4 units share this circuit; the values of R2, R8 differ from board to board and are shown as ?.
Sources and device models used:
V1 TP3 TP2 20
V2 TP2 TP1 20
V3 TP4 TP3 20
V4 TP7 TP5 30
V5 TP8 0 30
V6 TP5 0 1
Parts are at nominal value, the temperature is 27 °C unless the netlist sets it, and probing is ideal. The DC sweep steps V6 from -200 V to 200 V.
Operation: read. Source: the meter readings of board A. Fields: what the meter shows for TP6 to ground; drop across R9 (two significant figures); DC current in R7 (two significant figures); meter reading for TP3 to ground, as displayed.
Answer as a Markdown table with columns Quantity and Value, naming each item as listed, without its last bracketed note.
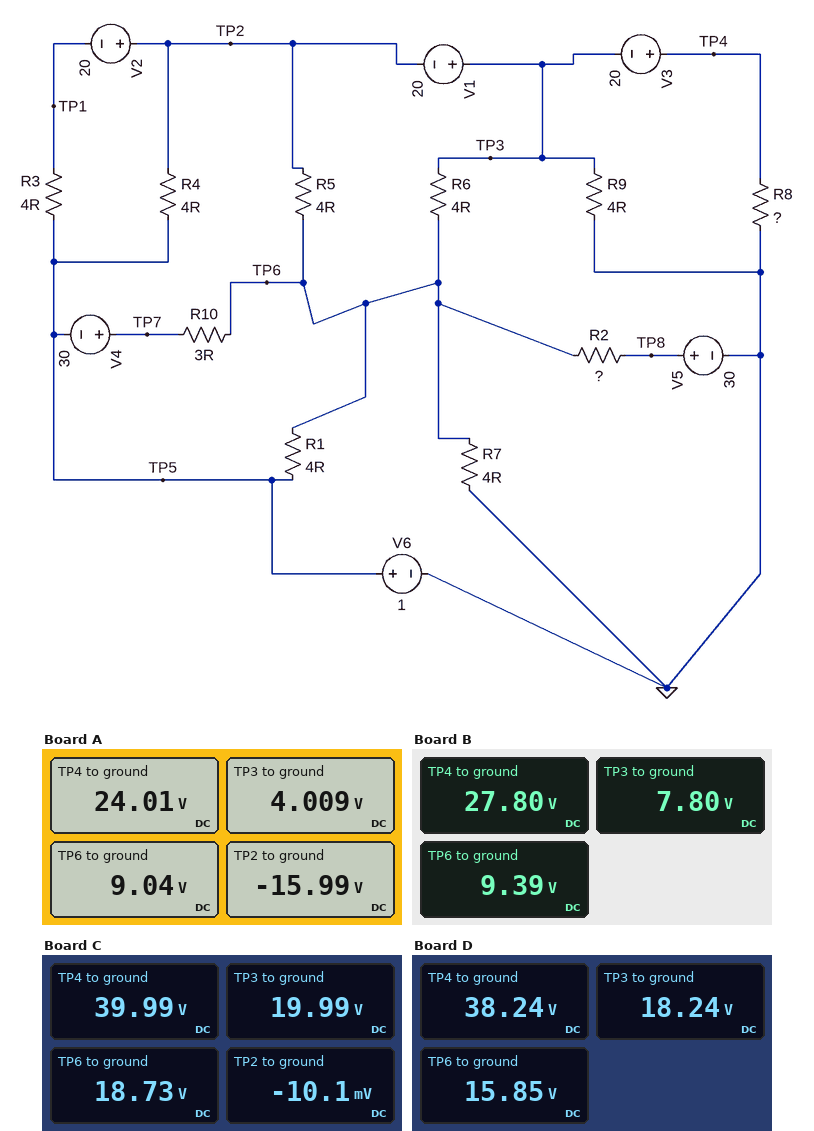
| Quantity | Value |
|---|---|
| what the meter shows for TP6 to ground | 9.04 V |
| drop across R9 | 4.0 V |
| DC current in R7 | 2.3 A |
| meter reading for TP3 to ground, as displayed | 4.009 V |
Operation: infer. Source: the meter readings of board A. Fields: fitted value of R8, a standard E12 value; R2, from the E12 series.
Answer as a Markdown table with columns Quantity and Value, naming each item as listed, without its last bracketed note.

| Quantity | Value |
|---|---|
| fitted value of R8, a standard E12 value | 1.2 Ω |
| R2, from the E12 series | 4.7 Ω |
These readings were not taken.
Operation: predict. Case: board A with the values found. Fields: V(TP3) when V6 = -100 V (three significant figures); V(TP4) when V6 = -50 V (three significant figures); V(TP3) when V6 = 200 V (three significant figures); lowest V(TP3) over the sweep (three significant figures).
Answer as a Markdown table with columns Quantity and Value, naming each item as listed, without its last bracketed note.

| Quantity | Value |
|---|---|
| V(TP3) when V6 = -100 V | -32.2 V |
| V(TP4) when V6 = -50 V | 5.73 V |
| V(TP3) when V6 = 200 V | 75.3 V |
| lowest V(TP3) over the sweep | -68.0 V |
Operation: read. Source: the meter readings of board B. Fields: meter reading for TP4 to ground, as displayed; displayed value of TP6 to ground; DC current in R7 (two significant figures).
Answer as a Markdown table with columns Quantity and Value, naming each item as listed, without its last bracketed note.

| Quantity | Value |
|---|---|
| meter reading for TP4 to ground, as displayed | 27.80 V |
| displayed value of TP6 to ground | 9.39 V |
| DC current in R7 | 2.3 A |
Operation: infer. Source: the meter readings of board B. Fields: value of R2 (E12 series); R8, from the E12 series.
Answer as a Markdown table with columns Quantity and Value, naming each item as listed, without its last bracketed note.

| Quantity | Value |
|---|---|
| value of R2 | 6.8 Ω |
| R8, from the E12 series | 1.8 Ω |
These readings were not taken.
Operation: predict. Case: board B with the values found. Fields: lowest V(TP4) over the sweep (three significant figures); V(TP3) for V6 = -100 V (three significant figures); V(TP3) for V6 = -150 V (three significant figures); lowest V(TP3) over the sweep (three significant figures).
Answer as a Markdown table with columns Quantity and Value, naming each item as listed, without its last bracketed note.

| Quantity | Value |
|---|---|
| lowest V(TP4) over the sweep | -57.8 V |
| V(TP3) for V6 = -100 V | -35.2 V |
| V(TP3) for V6 = -150 V | -56.5 V |
| lowest V(TP3) over the sweep | -77.8 V |
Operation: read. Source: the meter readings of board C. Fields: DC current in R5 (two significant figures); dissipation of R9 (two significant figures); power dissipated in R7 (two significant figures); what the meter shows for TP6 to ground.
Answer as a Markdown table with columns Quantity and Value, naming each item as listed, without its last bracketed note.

| Quantity | Value |
|---|---|
| DC current in R5 | 4.7 A |
| dissipation of R9 | 100 W |
| power dissipated in R7 | 88 W |
| what the meter shows for TP6 to ground | 18.73 V |
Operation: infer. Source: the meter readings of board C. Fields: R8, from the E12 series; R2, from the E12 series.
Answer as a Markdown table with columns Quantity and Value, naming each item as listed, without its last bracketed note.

| Quantity | Value |
|---|---|
| R8, from the E12 series | 8.2 Ω |
| R2, from the E12 series | 1.2 Ω |
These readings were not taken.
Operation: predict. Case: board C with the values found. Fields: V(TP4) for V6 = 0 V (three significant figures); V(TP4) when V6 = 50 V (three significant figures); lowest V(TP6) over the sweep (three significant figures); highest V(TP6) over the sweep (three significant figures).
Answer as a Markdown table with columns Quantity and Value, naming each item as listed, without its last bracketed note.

| Quantity | Value |
|---|---|
| V(TP4) for V6 = 0 V | 39.5 V |
| V(TP4) when V6 = 50 V | 64.7 V |
| lowest V(TP6) over the sweep | -58.8 V |
| highest V(TP6) over the sweep | 95.5 V |
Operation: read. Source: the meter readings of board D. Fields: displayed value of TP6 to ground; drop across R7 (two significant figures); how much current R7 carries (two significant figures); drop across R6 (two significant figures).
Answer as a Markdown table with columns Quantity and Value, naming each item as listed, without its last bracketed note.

| Quantity | Value |
|---|---|
| displayed value of TP6 to ground | 15.85 V |
| drop across R7 | 16 V |
| how much current R7 carries | 4.0 A |
| drop across R6 | 2.4 V |
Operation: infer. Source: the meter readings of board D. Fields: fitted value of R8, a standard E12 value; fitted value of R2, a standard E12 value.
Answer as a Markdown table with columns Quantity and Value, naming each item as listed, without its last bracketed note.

| Quantity | Value |
|---|---|
| fitted value of R8, a standard E12 value | 6.8 Ω |
| fitted value of R2, a standard E12 value | 2.2 Ω |
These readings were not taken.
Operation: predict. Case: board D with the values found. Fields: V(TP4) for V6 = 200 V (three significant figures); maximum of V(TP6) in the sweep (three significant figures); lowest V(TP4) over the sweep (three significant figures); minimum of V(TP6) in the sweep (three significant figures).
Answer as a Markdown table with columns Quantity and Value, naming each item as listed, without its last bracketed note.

| Quantity | Value |
|---|---|
| V(TP4) for V6 = 200 V | 143 V |
| maximum of V(TP6) in the sweep | 110 V |
| lowest V(TP4) over the sweep | -67.8 V |
| minimum of V(TP6) in the sweep | -79.4 V |
